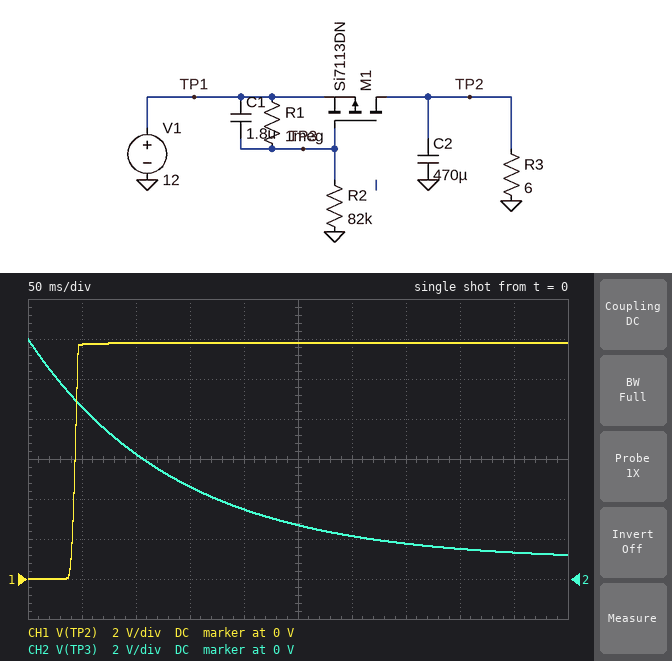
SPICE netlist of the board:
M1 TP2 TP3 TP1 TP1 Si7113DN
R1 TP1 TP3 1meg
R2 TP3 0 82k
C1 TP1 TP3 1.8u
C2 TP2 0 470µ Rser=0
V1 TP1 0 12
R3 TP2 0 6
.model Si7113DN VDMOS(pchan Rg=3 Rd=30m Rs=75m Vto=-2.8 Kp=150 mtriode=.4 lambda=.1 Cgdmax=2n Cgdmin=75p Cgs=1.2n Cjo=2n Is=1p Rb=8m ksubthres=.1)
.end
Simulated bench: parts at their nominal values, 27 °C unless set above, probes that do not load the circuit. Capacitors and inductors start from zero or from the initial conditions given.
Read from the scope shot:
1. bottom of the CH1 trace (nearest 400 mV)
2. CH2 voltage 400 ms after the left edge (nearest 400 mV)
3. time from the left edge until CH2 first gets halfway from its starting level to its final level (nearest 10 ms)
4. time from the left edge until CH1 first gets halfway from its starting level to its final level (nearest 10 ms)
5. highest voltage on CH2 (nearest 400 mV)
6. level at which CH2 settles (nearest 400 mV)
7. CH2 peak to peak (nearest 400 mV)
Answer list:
0 V
1.6 V
90 ms
40 ms
12.0 V
1.2 V
10.8 V
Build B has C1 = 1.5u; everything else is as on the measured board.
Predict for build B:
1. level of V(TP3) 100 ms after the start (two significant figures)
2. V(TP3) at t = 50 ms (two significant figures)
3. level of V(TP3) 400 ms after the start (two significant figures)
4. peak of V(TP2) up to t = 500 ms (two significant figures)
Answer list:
5.5 V
8.1 V
1.2 V
12 V
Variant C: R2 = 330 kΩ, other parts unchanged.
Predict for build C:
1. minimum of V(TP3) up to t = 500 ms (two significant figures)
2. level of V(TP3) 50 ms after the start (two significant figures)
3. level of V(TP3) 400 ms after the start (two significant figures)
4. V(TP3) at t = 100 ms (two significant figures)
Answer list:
5.9 V
11 V
6.7 V
10 V
